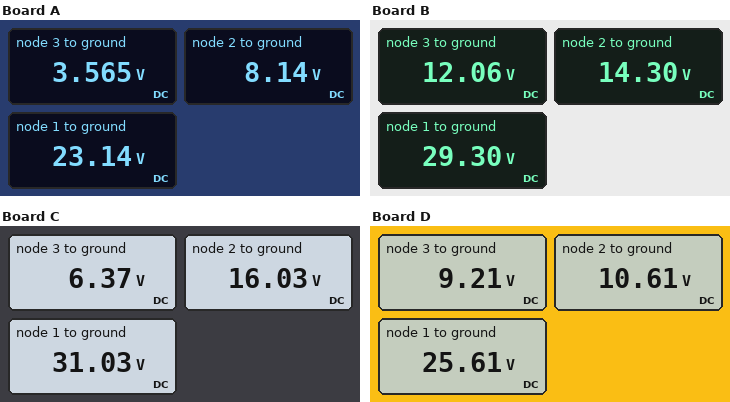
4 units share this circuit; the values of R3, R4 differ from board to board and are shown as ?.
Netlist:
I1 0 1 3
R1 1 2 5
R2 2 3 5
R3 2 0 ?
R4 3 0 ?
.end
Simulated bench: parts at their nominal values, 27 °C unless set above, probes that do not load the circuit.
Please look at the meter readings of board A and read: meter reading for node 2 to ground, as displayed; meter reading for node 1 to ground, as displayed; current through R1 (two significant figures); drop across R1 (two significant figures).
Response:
8.14 V
23.14 V
3.0 A
15 V
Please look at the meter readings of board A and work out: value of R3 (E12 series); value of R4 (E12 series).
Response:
3.9 Ω
3.9 Ω
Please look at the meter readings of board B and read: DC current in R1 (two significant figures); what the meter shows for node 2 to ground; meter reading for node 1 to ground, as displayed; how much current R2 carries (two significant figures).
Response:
3.0 A
14.30 V
29.30 V
450 mA
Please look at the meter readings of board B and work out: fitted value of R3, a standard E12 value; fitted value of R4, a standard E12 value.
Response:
5.6 Ω
27 Ω
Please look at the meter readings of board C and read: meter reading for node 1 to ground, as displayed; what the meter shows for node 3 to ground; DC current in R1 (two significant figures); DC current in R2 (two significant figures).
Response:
31.03 V
6.37 V
3.0 A
1.9 A
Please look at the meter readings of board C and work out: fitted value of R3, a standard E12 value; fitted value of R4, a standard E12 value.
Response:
15 Ω
3.3 Ω
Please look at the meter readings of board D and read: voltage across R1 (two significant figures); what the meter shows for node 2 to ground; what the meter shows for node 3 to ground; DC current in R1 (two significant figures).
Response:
15 V
10.61 V
9.21 V
3.0 A
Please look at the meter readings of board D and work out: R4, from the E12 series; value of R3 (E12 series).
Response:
33 Ω
3.9 Ω
